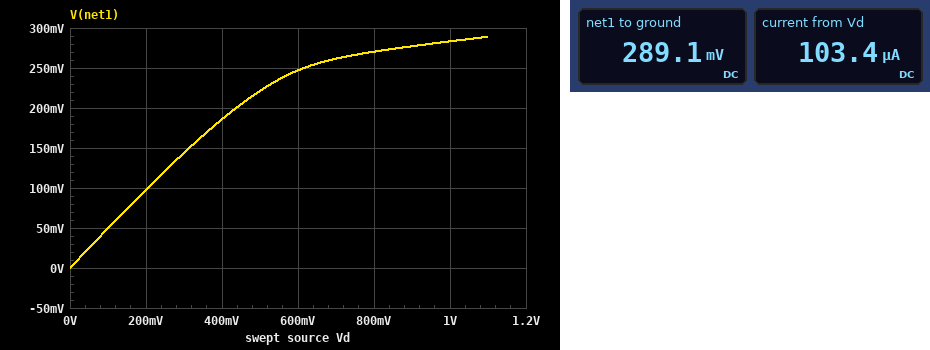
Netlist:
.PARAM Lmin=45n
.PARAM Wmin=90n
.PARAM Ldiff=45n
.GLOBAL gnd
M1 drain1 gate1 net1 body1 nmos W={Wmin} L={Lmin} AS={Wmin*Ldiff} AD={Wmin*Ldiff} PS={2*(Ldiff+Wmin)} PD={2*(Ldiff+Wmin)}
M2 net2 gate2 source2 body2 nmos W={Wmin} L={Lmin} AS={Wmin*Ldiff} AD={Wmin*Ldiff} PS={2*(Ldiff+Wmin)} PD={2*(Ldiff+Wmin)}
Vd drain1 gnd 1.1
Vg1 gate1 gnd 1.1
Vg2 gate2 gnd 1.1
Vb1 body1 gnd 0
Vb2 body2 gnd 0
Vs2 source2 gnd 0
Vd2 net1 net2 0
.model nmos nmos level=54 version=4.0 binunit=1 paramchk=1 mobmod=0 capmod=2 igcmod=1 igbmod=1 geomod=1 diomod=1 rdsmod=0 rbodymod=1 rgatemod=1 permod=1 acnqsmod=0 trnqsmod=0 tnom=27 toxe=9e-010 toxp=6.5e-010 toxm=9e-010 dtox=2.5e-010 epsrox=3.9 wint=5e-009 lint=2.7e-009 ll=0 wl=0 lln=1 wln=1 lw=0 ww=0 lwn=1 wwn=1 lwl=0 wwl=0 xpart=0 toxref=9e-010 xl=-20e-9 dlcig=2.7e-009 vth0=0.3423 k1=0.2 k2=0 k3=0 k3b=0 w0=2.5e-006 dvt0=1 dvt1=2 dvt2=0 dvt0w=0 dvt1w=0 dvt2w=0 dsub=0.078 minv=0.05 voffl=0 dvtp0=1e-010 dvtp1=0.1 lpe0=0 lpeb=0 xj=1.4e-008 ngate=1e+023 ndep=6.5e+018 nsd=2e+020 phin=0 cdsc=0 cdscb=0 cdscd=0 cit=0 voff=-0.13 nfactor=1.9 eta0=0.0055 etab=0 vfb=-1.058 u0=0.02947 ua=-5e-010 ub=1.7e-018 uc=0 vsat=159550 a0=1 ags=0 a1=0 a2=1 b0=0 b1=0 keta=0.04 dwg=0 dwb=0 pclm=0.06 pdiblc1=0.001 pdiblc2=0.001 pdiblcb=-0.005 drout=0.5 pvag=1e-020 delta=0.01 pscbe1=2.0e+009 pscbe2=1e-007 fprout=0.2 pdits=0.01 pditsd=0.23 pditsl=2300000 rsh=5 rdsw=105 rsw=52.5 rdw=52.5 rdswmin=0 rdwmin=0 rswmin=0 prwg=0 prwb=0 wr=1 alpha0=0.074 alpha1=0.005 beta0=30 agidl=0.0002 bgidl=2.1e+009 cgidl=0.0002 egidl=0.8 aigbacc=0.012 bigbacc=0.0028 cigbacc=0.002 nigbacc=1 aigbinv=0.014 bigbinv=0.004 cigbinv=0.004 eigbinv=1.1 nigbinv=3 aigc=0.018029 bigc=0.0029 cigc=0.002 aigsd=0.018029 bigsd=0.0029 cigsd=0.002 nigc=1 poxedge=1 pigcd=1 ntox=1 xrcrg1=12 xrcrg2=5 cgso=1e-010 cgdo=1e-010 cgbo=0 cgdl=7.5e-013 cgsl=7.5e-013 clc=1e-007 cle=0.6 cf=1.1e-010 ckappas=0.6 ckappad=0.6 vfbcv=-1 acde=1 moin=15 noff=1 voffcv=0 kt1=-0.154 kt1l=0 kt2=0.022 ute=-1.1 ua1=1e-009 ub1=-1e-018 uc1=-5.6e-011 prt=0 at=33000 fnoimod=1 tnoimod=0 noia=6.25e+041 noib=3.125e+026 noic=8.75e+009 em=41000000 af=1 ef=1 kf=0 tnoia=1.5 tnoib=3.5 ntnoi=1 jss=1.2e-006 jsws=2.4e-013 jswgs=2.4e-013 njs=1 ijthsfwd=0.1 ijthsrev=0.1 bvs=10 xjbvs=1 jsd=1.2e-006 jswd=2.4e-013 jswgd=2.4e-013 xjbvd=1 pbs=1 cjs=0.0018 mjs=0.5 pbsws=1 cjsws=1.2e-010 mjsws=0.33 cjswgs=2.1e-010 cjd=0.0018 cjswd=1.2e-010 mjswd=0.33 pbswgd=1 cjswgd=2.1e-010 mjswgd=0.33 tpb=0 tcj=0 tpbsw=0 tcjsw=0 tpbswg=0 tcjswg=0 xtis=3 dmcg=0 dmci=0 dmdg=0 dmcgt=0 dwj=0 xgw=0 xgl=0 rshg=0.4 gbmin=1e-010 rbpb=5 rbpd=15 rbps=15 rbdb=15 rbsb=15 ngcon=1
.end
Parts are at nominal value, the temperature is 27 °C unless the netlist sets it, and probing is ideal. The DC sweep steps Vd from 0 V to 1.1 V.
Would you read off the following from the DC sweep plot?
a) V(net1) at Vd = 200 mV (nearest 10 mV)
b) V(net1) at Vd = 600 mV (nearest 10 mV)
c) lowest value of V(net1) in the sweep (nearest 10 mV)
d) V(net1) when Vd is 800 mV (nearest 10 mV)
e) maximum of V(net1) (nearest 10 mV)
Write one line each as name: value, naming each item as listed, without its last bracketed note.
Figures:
V(net1) at Vd = 200 mV: 100 mV
V(net1) at Vd = 600 mV: 250 mV
lowest value of V(net1) in the sweep: 0 V
V(net1) when Vd is 800 mV: 270 mV
maximum of V(net1): 290 mV
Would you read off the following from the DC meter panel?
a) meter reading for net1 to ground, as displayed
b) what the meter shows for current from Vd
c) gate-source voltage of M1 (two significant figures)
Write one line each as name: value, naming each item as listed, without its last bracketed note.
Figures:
meter reading for net1 to ground, as displayed: 289.1 mV
what the meter shows for current from Vd: 103.4 µA
gate-source voltage of M1: 810 mV
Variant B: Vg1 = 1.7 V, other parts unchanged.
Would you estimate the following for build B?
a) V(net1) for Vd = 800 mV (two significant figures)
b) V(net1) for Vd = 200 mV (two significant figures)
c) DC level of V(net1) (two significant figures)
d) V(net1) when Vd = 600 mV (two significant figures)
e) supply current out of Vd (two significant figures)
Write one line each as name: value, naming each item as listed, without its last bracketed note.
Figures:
V(net1) for Vd = 800 mV: 410 mV
V(net1) for Vd = 200 mV: 100 mV
DC level of V(net1): 530 mV
V(net1) when Vd = 600 mV: 310 mV
supply current out of Vd: 150 µA
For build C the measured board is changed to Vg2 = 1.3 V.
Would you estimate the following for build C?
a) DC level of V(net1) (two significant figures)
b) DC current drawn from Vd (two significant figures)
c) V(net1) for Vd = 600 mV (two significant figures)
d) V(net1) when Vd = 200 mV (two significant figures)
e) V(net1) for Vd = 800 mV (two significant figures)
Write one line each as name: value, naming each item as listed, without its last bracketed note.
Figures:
DC level of V(net1): 280 mV
DC current drawn from Vd: 110 µA
V(net1) for Vd = 600 mV: 240 mV
V(net1) when Vd = 200 mV: 97 mV
V(net1) for Vd = 800 mV: 260 mV
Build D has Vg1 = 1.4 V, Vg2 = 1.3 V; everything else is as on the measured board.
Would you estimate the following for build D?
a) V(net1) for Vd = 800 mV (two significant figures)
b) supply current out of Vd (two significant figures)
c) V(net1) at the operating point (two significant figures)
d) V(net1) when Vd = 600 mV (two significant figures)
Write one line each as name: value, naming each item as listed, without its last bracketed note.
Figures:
V(net1) for Vd = 800 mV: 350 mV
supply current out of Vd: 140 µA
V(net1) at the operating point: 390 mV
V(net1) when Vd = 600 mV: 280 mV
